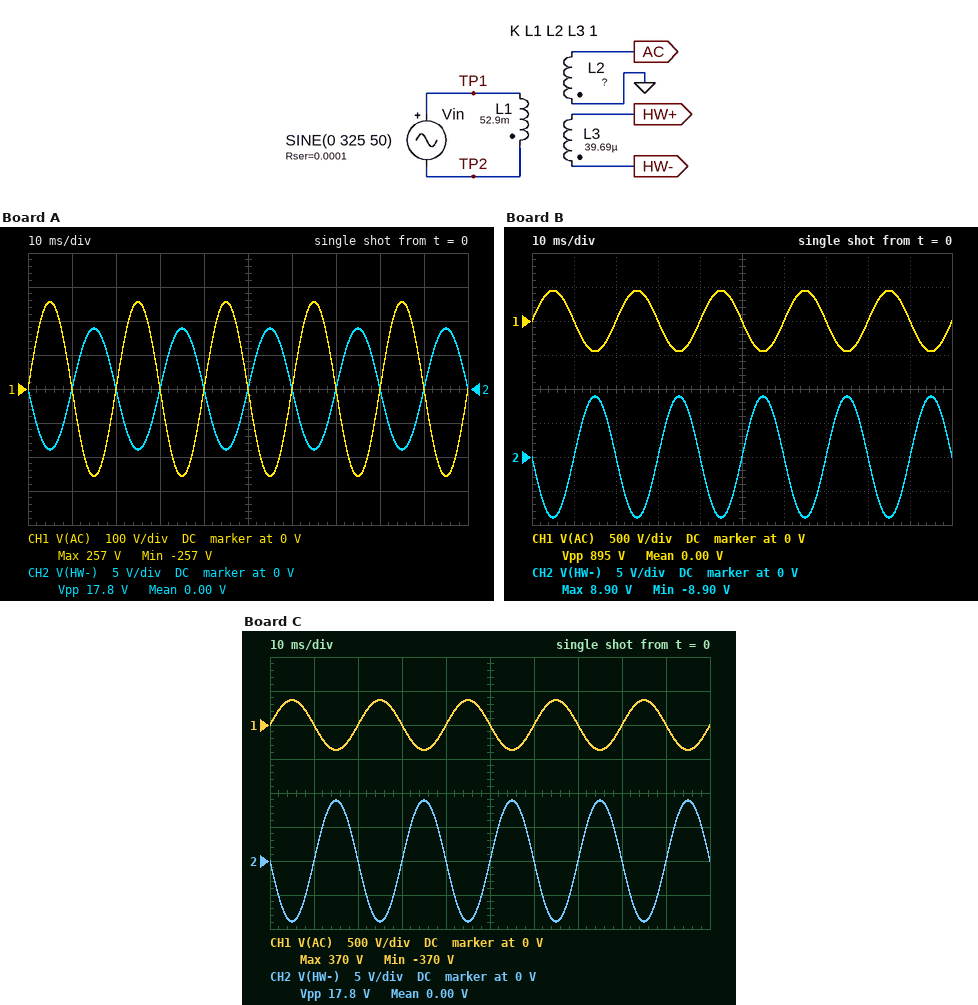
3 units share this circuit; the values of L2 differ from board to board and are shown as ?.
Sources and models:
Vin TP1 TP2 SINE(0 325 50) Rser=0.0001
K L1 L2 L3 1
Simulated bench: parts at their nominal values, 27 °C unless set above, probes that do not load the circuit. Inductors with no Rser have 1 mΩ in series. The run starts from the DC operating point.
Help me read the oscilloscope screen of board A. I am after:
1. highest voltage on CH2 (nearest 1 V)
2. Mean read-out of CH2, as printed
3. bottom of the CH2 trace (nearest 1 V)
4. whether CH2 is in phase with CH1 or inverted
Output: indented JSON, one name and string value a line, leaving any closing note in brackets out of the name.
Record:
{
  "highest voltage on CH2": "9 V",
  "Mean read-out of CH2, as printed": "0.00 V",
  "bottom of the CH2 trace": "-9 V",
  "whether CH2 is in phase with CH1 or inverted": "inverted"
}
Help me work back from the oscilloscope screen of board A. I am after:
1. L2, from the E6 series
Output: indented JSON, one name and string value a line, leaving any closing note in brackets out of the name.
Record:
{
  "L2, from the E6 series": "33 mH"
}
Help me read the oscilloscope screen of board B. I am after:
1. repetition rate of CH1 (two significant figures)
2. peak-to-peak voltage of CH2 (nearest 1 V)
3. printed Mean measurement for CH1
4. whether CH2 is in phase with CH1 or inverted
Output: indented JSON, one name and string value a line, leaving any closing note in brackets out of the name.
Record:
{
  "repetition rate of CH1": "50 Hz",
  "peak-to-peak voltage of CH2": "18 V",
  "printed Mean measurement for CH1": "0.00 V",
  "whether CH2 is in phase with CH1 or inverted": "inverted"
}
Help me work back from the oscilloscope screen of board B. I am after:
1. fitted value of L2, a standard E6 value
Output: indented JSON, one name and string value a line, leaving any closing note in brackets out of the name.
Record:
{
  "fitted value of L2, a standard E6 value": "100 mH"
}
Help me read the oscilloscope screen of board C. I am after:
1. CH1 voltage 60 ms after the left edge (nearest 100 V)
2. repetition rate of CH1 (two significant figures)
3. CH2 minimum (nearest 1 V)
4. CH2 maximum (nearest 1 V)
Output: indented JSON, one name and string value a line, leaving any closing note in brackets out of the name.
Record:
{
  "CH1 voltage 60 ms after the left edge": "0 V",
  "repetition rate of CH1": "50 Hz",
  "CH2 minimum": "-9 V",
  "CH2 maximum": "9 V"
}
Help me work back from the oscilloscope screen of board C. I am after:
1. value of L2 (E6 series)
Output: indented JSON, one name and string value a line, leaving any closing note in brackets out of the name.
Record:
{
  "value of L2": "68 mH"
}
